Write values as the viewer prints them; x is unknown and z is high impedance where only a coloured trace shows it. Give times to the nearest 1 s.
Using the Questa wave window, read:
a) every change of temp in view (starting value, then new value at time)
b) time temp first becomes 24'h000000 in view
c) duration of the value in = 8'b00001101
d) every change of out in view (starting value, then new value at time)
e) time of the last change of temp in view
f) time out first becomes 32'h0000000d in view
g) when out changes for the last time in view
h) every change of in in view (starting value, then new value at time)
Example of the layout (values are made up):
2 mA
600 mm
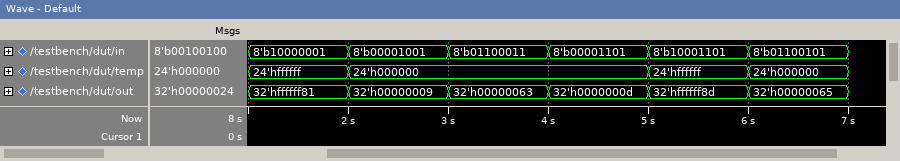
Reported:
24'hffffff, 24'h000000 at 2 s, 24'hffffff at 5 s, 24'h000000 at 6 s
2 s
1 s
32'hffffff81, 32'h00000009 at 2 s, 32'h00000063 at 3 s, 32'h0000000d at 4 s, 32'hffffff8d at 5 s, 32'h00000065 at 6 s
6 s
4 s
6 s
8'b10000001, 8'b00001001 at 2 s, 8'b01100011 at 3 s, 8'b00001101 at 4 s, 8'b10001101 at 5 s, 8'b01100101 at 6 s
